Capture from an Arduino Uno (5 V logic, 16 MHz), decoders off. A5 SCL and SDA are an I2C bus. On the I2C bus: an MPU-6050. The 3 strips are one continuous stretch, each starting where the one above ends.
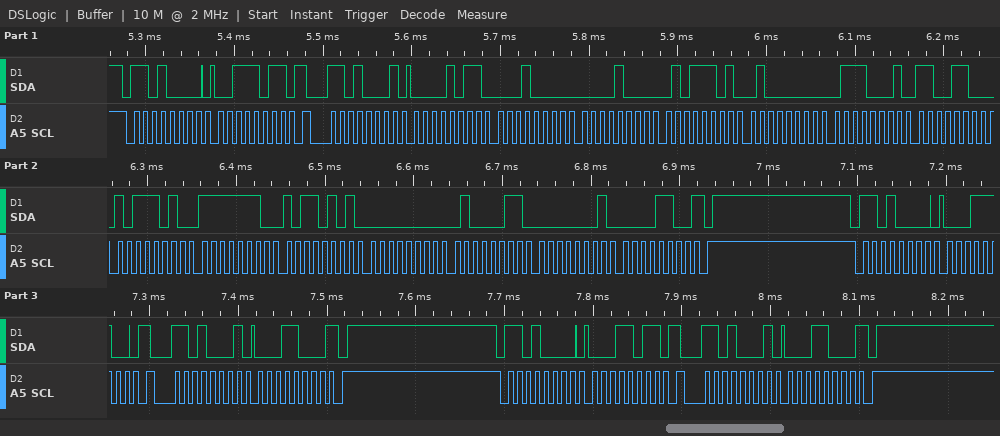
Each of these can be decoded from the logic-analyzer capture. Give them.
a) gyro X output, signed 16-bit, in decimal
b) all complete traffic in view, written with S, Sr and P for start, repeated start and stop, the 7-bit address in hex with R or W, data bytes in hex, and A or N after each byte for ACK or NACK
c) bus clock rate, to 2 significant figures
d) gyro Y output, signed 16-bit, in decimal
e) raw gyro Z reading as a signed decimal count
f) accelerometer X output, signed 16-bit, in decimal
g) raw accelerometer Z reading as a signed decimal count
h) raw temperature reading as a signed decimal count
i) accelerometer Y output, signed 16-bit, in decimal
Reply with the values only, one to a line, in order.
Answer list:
-331
S 68W A 3B A Sr 68R A 0B A 10 A 08 A 5D A 40 A 71 A CC A BA A FE A B5 A 00 A 43 A 01 A 0C N P S 68W A 1C A Sr 68R A 18 N P S 68W A 1B A Sr 68R A 18 N P
100 kHz
67
268
2832
16497
-13126
2141
